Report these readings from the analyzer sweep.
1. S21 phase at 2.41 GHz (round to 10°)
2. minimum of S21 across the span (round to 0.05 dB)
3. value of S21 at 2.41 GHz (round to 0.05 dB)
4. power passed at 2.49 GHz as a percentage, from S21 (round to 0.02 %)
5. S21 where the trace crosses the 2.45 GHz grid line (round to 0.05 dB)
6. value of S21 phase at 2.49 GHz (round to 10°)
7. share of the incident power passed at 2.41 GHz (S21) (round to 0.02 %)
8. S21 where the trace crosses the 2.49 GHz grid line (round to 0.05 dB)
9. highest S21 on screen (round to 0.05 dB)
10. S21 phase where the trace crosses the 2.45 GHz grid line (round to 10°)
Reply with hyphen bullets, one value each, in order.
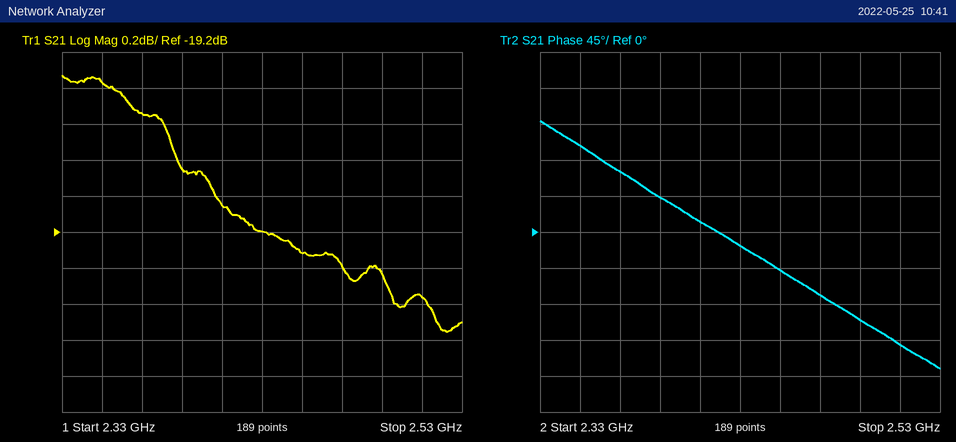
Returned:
- 10°
- -19.75 dB
- -19.05 dB
- 1.14 %
- -19.30 dB
- -110°
- 1.24 %
- -19.45 dB
- -18.35 dB
- -50°
